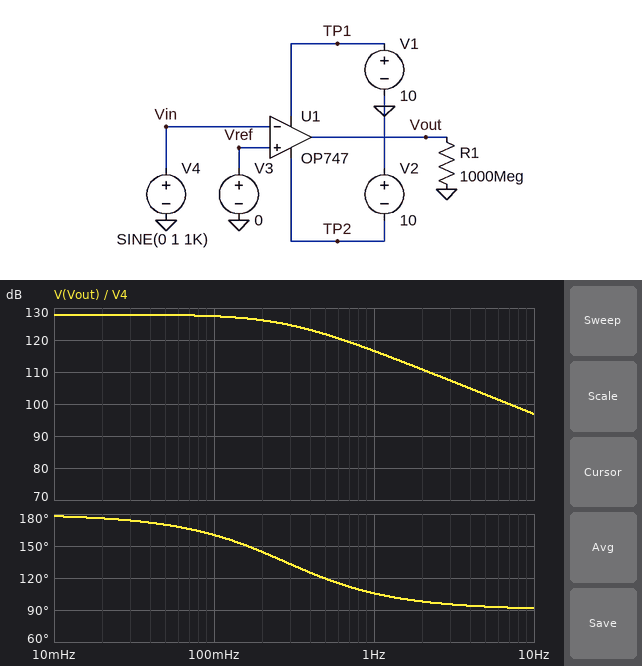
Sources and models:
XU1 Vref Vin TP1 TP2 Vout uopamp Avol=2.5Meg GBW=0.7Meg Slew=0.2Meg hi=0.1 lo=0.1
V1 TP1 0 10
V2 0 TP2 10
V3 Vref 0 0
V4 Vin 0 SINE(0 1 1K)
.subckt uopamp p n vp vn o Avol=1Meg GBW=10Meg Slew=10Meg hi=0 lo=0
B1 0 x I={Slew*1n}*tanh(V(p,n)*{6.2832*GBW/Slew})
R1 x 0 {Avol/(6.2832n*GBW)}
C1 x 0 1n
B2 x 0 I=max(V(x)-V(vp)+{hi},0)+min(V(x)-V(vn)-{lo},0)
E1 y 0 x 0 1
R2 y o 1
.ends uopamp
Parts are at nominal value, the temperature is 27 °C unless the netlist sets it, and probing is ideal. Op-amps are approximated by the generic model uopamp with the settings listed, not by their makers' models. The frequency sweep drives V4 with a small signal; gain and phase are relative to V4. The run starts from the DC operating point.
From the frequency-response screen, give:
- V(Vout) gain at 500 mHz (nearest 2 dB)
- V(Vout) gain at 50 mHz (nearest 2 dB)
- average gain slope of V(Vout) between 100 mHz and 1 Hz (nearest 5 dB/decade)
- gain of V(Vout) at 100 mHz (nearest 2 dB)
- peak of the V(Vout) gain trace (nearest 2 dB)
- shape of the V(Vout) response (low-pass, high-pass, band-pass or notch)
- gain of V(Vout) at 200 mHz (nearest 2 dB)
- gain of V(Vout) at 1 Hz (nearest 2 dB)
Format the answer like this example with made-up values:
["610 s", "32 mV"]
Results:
["122 dB", "128 dB", "-10 dB/decade", "128 dB", "128 dB", "low-pass", "126 dB", "116 dB"]
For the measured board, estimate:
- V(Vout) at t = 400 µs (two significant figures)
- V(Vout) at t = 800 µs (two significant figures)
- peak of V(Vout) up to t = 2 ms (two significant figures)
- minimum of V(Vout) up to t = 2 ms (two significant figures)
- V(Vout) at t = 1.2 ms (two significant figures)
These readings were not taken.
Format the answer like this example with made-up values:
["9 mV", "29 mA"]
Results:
["-9.9 V", "9.9 V", "9.9 V", "-9.9 V", "-9.9 V"]
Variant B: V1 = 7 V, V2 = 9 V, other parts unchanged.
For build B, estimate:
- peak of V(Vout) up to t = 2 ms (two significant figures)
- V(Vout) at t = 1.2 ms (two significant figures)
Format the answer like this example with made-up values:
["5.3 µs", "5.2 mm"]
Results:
["6.9 V", "-8.9 V"]
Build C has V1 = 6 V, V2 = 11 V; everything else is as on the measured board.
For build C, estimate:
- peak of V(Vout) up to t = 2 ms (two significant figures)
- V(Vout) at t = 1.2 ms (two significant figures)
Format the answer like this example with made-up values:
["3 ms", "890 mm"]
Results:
["5.9 V", "-11 V"]
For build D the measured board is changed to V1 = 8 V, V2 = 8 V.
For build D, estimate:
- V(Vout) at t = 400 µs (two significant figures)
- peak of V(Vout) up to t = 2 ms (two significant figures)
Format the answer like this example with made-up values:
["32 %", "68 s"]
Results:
["-7.9 V", "7.9 V"]
